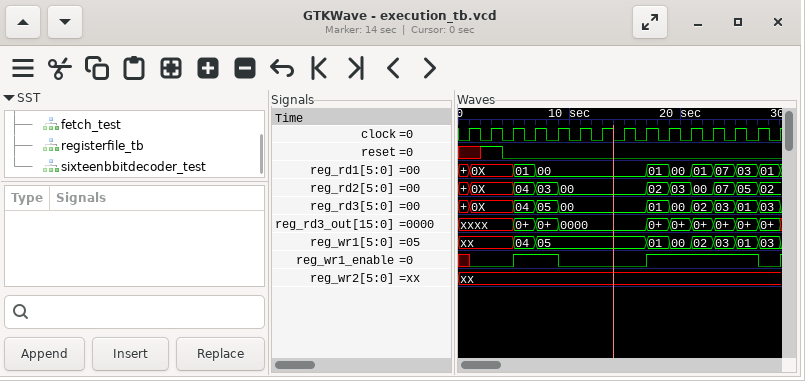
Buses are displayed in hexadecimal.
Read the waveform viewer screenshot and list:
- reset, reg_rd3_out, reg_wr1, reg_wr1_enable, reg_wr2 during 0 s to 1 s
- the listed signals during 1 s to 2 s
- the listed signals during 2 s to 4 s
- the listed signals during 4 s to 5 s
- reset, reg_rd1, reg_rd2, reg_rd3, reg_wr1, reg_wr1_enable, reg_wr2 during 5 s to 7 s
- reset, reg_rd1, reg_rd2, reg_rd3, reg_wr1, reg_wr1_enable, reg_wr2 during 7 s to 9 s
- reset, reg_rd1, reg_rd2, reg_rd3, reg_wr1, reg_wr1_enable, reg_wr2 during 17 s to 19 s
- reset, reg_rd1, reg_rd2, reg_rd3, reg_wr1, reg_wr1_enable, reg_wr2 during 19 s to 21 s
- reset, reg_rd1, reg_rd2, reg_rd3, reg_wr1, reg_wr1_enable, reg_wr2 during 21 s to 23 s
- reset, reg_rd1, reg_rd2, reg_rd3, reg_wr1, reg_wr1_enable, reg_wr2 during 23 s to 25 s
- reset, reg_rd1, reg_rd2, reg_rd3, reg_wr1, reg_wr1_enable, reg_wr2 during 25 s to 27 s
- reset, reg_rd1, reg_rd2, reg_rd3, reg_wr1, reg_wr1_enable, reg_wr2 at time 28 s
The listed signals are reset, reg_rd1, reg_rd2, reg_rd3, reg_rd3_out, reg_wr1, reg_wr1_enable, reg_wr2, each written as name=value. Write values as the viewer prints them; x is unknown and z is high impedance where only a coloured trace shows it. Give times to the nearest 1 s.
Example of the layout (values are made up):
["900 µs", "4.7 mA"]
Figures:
["reset=x, reg_rd3_out=xxxx, reg_wr1=xx, reg_wr1_enable=x, reg_wr2=xx", "reset=x, reg_rd1=0X, reg_rd2=0X, reg_rd3=0X, reg_rd3_out=xxxx, reg_wr1=xx, reg_wr1_enable=0, reg_wr2=xx", "reset=1, reg_rd1=0X, reg_rd2=0X, reg_rd3=0X, reg_rd3_out=xxxx, reg_wr1=xx, reg_wr1_enable=0, reg_wr2=xx", "reset=0, reg_rd1=0X, reg_rd2=0X, reg_rd3=0X, reg_rd3_out=xxxx, reg_wr1=xx, reg_wr1_enable=0, reg_wr2=xx", "reset=0, reg_rd1=01, reg_rd2=04, reg_rd3=04, reg_wr1=04, reg_wr1_enable=1, reg_wr2=xx", "reset=0, reg_rd1=00, reg_rd2=03, reg_rd3=05, reg_wr1=05, reg_wr1_enable=1, reg_wr2=xx", "reset=0, reg_rd1=01, reg_rd2=02, reg_rd3=01, reg_wr1=01, reg_wr1_enable=1, reg_wr2=xx", "reset=0, reg_rd1=00, reg_rd2=03, reg_rd3=00, reg_wr1=00, reg_wr1_enable=1, reg_wr2=xx", "reset=0, reg_rd1=01, reg_rd2=00, reg_rd3=02, reg_wr1=02, reg_wr1_enable=1, reg_wr2=xx", "reset=0, reg_rd1=07, reg_rd2=07, reg_rd3=03, reg_wr1=03, reg_wr1_enable=1, reg_wr2=xx", "reset=0, reg_rd1=03, reg_rd2=05, reg_rd3=01, reg_wr1=01, reg_wr1_enable=1, reg_wr2=xx", "reset=0, reg_rd1=01, reg_rd2=02, reg_rd3=03, reg_wr1=03, reg_wr1_enable=0, reg_wr2=xx"]
